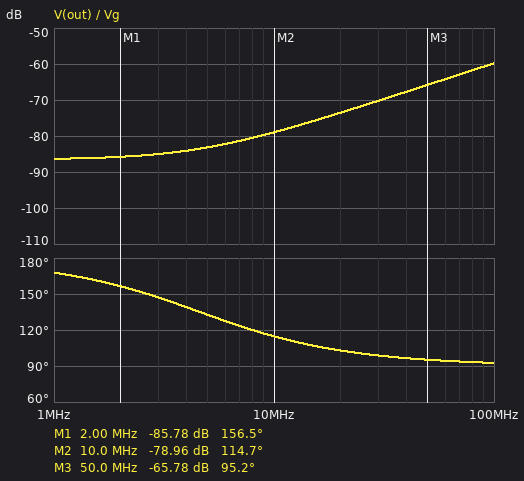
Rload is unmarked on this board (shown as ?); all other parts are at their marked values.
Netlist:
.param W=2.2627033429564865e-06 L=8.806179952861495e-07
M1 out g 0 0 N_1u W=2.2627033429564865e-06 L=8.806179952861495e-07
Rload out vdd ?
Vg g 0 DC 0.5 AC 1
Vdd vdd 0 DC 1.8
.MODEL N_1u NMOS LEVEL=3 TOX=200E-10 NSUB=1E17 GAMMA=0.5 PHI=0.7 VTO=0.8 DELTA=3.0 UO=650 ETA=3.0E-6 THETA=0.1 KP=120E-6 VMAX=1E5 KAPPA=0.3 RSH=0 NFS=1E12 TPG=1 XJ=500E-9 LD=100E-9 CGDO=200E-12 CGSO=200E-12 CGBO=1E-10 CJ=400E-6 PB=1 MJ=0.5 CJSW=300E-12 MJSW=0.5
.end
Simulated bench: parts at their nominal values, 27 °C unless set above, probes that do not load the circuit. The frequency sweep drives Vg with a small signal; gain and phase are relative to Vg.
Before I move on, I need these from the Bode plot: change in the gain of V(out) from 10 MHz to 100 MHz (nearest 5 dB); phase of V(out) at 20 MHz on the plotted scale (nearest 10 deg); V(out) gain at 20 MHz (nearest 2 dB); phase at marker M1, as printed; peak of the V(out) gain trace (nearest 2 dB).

20 dB
100 deg
-74 dB
156.5 deg
-60 dB
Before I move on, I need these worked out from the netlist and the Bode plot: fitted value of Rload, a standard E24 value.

3.6 kΩ
